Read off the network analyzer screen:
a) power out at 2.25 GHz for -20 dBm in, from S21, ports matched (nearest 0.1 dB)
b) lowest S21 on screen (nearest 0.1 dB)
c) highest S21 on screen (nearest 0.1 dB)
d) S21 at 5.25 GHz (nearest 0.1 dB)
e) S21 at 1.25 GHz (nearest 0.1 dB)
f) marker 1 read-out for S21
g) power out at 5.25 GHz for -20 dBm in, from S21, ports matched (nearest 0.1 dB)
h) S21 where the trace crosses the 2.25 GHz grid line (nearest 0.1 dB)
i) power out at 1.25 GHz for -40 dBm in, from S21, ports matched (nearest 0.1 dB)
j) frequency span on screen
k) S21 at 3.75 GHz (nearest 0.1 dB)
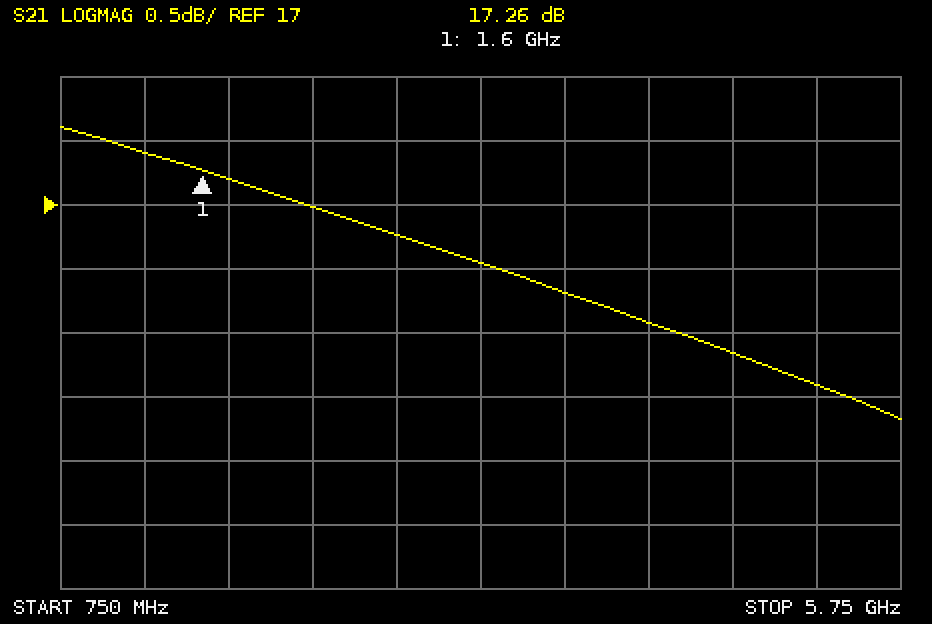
-3.0 dBm
15.3 dB
17.6 dB
15.6 dB
17.4 dB
17.26 dB
-4.4 dBm
17.0 dB
-22.6 dBm
5 GHz
16.3 dB
